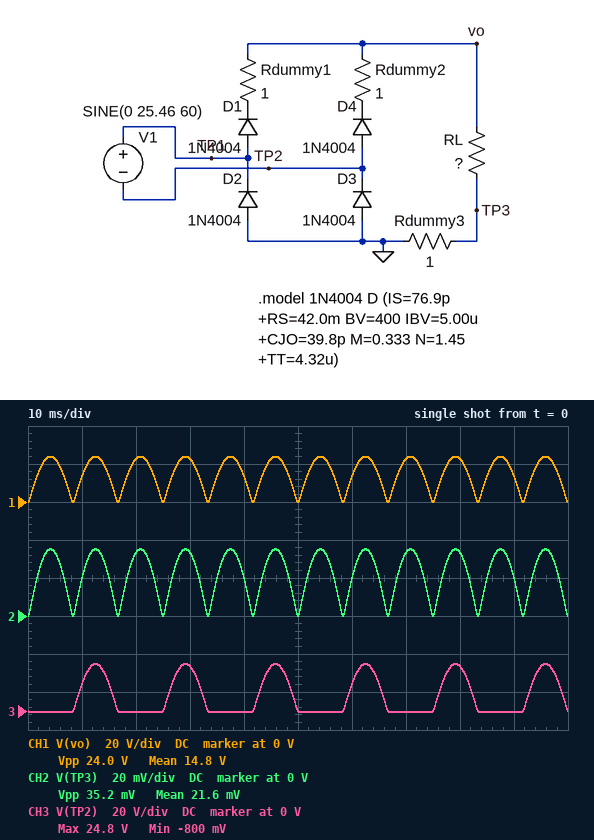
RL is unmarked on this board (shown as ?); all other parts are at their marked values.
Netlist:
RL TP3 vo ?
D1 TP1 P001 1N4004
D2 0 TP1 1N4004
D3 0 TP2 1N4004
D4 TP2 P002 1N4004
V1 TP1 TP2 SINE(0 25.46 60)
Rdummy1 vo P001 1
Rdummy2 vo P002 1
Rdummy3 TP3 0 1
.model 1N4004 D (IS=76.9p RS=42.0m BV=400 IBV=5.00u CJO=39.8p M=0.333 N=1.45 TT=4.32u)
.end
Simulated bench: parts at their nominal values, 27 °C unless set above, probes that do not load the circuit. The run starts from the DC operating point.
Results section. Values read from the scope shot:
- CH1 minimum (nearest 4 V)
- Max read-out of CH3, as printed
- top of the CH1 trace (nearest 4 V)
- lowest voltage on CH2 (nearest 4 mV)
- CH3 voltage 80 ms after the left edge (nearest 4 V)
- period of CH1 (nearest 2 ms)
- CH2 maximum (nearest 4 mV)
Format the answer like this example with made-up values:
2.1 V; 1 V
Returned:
0 V; 24.8 V; 24 V; 0 V; 24 V; 8 ms; 36 mV
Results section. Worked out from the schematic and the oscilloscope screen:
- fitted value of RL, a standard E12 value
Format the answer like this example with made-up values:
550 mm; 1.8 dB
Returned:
680 Ω
